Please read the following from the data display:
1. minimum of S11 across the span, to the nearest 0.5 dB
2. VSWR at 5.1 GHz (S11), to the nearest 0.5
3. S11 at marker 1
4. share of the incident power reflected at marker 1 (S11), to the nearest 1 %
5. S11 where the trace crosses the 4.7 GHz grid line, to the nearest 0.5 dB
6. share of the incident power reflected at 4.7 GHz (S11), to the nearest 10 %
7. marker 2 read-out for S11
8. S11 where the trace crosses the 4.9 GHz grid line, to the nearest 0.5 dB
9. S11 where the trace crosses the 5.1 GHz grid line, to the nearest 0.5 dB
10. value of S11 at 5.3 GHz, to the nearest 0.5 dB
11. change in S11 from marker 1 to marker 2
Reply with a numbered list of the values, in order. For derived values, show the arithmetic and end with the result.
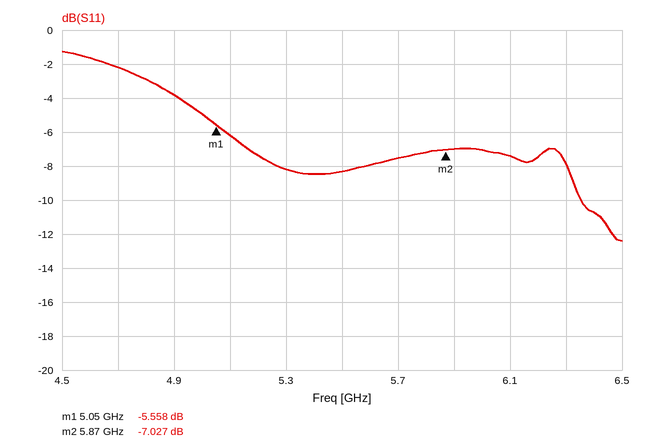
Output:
1. -12.5 dB
2. |Γ| = 10^(-6/20) = 0.5012; VSWR = (1 + 0.5012)/(1 − 0.5012) ≈ 3.0
3. -5.558 dB
4. 10^(-5.558/10) ≈ 28 %
5. -2.0 dB
6. 10^(-2/10) ≈ 63.1 %, so 60 % to the nearest 10 %
7. -7.027 dB
8. -4.0 dB
9. -6.0 dB
10. -8.0 dB
11. -7.027 − (-5.558) = -1.469 dB
